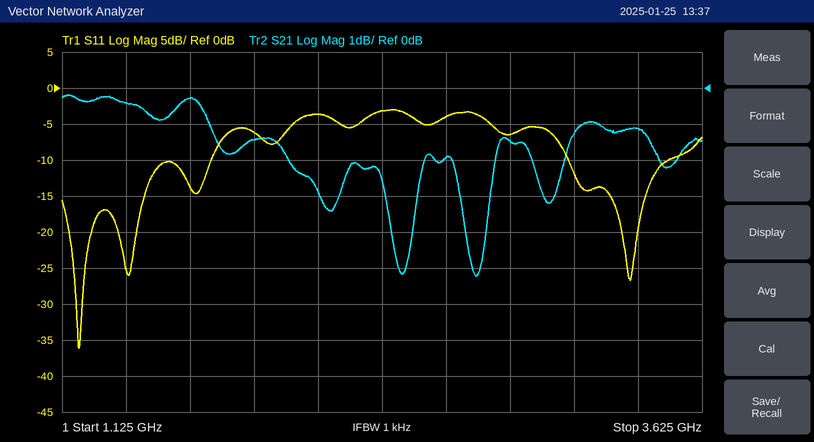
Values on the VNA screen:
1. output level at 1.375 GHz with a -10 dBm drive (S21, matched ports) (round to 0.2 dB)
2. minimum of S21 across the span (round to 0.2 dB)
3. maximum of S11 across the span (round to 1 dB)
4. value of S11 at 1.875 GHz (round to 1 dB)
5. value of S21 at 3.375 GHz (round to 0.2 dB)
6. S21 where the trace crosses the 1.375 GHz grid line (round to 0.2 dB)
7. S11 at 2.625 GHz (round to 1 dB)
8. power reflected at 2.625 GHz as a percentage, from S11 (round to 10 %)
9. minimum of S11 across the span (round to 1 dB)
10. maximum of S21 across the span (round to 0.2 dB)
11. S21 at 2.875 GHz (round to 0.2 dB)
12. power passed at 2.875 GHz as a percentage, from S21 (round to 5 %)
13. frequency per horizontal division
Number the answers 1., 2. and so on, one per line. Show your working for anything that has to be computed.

1. -10 dBm + (-0.4 dB) = -10.4 dBm
2. -5.2 dB
3. -3 dB
4. -6 dB
5. -1.2 dB
6. -0.4 dB
7. -4 dB
8. 10^(-4/10) ≈ 40 %
9. -36 dB
10. -0.2 dB
11. -1.4 dB
12. 10^(-1.4/10) ≈ 72.4 %, so 70 % to the nearest 5 %
13. 250 MHz
